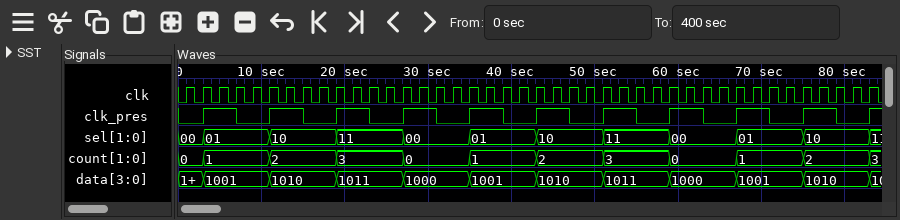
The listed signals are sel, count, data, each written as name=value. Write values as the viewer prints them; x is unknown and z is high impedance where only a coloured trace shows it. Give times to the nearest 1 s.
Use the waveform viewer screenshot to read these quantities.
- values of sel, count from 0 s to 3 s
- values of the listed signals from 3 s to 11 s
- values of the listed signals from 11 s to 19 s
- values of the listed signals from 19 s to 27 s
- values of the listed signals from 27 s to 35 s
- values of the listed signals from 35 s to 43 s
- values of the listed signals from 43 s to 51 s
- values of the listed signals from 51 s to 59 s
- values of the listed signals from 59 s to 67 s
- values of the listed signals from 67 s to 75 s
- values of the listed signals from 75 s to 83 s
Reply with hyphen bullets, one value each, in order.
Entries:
- sel=00, count=0
- sel=01, count=1, data=1001
- sel=10, count=2, data=1010
- sel=11, count=3, data=1011
- sel=00, count=0, data=1000
- sel=01, count=1, data=1001
- sel=10, count=2, data=1010
- sel=11, count=3, data=1011
- sel=00, count=0, data=1000
- sel=01, count=1, data=1001
- sel=10, count=2, data=1010
